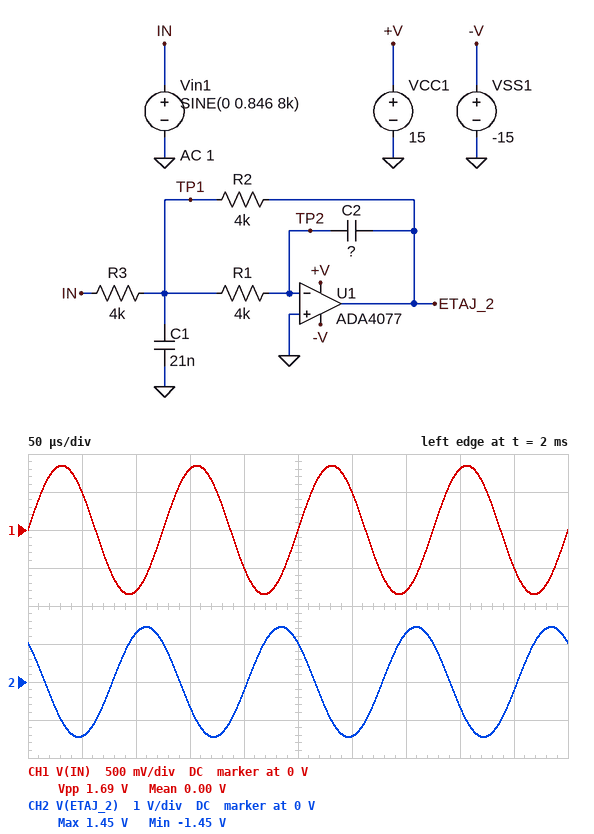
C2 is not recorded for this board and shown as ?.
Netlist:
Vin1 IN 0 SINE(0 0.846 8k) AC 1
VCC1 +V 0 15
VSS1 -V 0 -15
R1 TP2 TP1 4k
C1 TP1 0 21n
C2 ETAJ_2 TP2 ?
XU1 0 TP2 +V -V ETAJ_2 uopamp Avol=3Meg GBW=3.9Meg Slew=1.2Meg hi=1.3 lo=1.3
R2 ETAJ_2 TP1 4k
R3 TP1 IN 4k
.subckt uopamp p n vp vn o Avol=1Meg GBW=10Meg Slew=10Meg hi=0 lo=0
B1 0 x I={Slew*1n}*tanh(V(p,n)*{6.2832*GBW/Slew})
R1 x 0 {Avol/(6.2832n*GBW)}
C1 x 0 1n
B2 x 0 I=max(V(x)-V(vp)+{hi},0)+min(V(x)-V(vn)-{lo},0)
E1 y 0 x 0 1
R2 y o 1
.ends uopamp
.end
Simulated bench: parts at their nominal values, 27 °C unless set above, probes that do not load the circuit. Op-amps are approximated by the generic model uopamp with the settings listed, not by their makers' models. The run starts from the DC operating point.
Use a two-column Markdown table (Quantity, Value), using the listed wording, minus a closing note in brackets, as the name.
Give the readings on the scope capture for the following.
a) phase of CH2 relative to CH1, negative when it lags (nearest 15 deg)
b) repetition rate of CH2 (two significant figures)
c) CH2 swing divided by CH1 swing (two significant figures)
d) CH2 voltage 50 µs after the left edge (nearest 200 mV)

| Quantity | Value |
|---|---|
| phase of CH2 relative to CH1, negative when it lags | 135 deg |
| repetition rate of CH2 | 8.0 kHz |
| CH2 swing divided by CH1 swing | 1.7 |
| CH2 voltage 50 µs after the left edge | -1.4 V |
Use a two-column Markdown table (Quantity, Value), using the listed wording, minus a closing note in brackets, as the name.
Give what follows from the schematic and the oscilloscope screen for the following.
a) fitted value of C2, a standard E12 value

| Quantity | Value |
|---|---|
| fitted value of C2, a standard E12 value | 680 pF |
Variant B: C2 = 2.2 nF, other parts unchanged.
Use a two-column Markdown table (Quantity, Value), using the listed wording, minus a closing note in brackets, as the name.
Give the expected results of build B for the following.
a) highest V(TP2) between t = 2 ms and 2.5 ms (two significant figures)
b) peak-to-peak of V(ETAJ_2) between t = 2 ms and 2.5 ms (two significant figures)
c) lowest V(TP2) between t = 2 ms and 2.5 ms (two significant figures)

| Quantity | Value |
|---|---|
| highest V(TP2) between t = 2 ms and 2.5 ms | 1.1 mV |
| peak-to-peak of V(ETAJ_2) between t = 2 ms and 2.5 ms | 1.1 V |
| lowest V(TP2) between t = 2 ms and 2.5 ms | -1.1 mV |
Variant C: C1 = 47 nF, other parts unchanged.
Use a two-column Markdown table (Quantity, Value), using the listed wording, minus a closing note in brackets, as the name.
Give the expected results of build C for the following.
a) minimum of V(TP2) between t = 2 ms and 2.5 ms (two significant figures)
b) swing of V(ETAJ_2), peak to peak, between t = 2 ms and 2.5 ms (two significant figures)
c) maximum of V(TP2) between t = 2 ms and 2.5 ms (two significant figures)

| Quantity | Value |
|---|---|
| minimum of V(TP2) between t = 2 ms and 2.5 ms | -3.4 mV |
| swing of V(ETAJ_2), peak to peak, between t = 2 ms and 2.5 ms | 3.3 V |
| maximum of V(TP2) between t = 2 ms and 2.5 ms | 3.4 mV |
